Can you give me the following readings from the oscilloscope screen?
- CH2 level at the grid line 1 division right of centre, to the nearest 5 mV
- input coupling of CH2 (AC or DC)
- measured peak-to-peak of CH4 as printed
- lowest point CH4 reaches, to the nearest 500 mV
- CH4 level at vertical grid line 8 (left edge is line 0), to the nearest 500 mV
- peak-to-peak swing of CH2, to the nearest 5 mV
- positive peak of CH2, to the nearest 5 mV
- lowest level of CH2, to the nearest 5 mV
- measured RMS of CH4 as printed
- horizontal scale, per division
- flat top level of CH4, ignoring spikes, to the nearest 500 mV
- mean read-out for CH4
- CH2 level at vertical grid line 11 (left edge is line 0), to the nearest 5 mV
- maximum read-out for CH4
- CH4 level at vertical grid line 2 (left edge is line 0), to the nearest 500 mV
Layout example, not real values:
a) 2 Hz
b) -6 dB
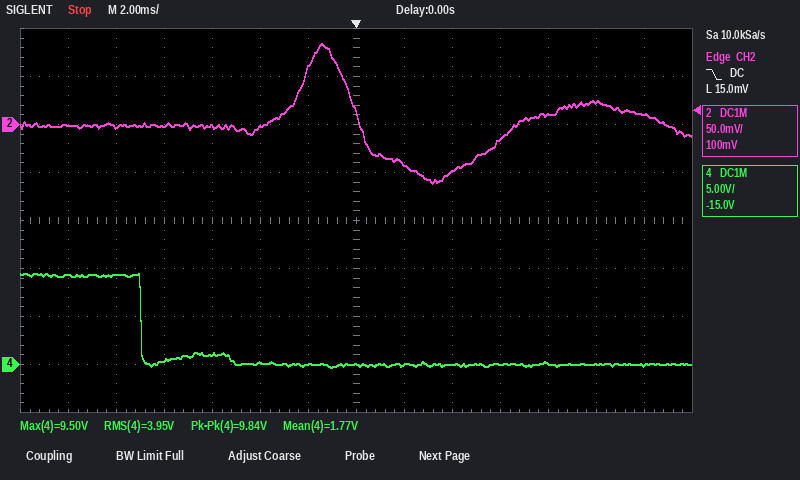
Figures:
a) -40 mV
b) DC
c) 9.84 V
d) -500 mV
e) 0.0 V
f) 145 mV
g) 85 mV
h) -60 mV
i) 3.95 V
j) 2 ms
k) 9.5 V
l) 1.77 V
m) 10 mV
n) 9.50 V
o) 9.5 V
